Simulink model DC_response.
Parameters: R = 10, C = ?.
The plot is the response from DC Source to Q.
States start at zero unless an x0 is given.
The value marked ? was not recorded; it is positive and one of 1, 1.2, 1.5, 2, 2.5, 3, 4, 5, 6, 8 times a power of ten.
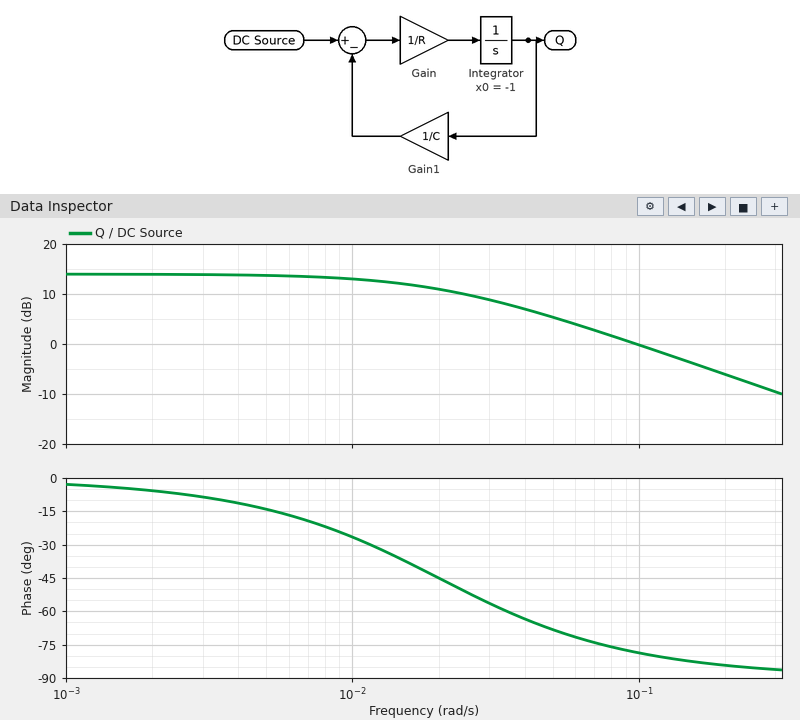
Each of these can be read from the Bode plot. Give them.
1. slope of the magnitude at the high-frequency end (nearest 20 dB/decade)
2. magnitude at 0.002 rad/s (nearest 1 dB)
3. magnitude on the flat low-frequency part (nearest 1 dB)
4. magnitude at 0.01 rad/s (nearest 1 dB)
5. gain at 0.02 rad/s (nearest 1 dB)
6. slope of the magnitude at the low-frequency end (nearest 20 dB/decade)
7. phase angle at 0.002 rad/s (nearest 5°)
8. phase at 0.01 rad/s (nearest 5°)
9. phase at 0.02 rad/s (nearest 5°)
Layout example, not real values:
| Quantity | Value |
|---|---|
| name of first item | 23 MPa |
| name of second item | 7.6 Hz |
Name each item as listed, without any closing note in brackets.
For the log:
| Quantity | Value |
|---|---|
| slope of the magnitude at the high-frequency end | -20 dB/decade |
| magnitude at 0.002 rad/s | 14 dB |
| magnitude on the flat low-frequency part | 14 dB |
| magnitude at 0.01 rad/s | 13 dB |
| gain at 0.02 rad/s | 11 dB |
| slope of the magnitude at the low-frequency end | 0 dB/decade |
| phase angle at 0.002 rad/s | -5° |
| phase at 0.01 rad/s | -25° |
| phase at 0.02 rad/s | -45° |
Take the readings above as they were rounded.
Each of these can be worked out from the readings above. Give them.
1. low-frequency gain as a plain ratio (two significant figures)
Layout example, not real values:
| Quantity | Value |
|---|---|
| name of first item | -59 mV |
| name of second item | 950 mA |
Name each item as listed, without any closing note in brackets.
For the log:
| Quantity | Value |
|---|---|
| low-frequency gain as a plain ratio | 5.0 |
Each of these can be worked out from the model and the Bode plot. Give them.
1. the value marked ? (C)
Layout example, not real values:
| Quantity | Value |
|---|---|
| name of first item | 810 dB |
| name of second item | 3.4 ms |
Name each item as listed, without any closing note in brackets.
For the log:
| Quantity | Value |
|---|---|
| the value marked ? | 5 |
